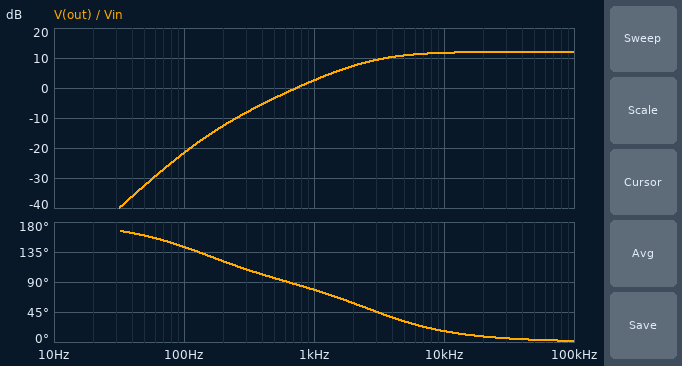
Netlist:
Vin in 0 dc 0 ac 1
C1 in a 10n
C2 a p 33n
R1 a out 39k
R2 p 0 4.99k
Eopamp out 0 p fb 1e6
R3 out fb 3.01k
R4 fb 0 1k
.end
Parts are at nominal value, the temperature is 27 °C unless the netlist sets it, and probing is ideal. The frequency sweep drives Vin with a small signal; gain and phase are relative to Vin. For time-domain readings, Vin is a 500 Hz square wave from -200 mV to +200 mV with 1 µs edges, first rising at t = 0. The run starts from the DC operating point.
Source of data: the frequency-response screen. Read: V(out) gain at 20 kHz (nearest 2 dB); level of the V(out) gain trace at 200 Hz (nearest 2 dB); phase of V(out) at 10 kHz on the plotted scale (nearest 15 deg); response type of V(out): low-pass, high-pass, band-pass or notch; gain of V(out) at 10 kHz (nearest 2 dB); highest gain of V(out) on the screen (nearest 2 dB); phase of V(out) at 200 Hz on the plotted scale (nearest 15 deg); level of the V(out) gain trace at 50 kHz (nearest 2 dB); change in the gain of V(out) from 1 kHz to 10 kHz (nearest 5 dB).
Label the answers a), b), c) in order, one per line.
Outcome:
a) 12 dB
b) -12 dB
c) 15 deg
d) high-pass
e) 12 dB
f) 12 dB
g) 120 deg
h) 12 dB
i) 10 dB
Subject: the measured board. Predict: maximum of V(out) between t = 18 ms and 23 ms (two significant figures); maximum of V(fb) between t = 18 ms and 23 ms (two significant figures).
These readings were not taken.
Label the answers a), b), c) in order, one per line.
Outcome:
a) 1.6 V
b) 400 mV
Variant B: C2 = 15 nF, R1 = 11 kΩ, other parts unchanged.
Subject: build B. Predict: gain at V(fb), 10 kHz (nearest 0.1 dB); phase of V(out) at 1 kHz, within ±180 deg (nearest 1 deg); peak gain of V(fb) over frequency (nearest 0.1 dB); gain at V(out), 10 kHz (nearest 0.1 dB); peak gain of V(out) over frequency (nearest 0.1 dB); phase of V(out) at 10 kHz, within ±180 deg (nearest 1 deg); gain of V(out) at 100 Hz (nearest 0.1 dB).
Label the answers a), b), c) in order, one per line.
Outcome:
a) 0.2 dB
b) 155 deg
c) 5.6 dB
d) 12.3 dB
e) 17.6 dB
f) 6 deg
g) -37.7 dB
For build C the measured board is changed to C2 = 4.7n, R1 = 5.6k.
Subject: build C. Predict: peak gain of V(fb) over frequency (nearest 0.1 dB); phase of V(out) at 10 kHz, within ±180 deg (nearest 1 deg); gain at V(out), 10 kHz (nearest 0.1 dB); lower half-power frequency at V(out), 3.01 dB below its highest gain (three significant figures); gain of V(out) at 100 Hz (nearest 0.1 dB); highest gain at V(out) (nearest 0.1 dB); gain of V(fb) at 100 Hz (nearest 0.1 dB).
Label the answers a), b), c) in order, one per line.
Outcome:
a) 9.9 dB
b) 10 deg
c) 13.8 dB
d) 3.90 kHz
e) -53.6 dB
f) 22.0 dB
g) -65.7 dB
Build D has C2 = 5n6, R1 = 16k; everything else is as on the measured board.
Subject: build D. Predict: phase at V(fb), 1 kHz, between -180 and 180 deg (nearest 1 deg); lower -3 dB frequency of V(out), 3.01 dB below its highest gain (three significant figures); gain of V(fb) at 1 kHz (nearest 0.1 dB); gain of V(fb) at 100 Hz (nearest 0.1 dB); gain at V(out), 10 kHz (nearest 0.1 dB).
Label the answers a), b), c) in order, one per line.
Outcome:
a) 128 deg
b) 4.97 kHz
c) -17.5 dB
d) -55.1 dB
e) 11.1 dB
